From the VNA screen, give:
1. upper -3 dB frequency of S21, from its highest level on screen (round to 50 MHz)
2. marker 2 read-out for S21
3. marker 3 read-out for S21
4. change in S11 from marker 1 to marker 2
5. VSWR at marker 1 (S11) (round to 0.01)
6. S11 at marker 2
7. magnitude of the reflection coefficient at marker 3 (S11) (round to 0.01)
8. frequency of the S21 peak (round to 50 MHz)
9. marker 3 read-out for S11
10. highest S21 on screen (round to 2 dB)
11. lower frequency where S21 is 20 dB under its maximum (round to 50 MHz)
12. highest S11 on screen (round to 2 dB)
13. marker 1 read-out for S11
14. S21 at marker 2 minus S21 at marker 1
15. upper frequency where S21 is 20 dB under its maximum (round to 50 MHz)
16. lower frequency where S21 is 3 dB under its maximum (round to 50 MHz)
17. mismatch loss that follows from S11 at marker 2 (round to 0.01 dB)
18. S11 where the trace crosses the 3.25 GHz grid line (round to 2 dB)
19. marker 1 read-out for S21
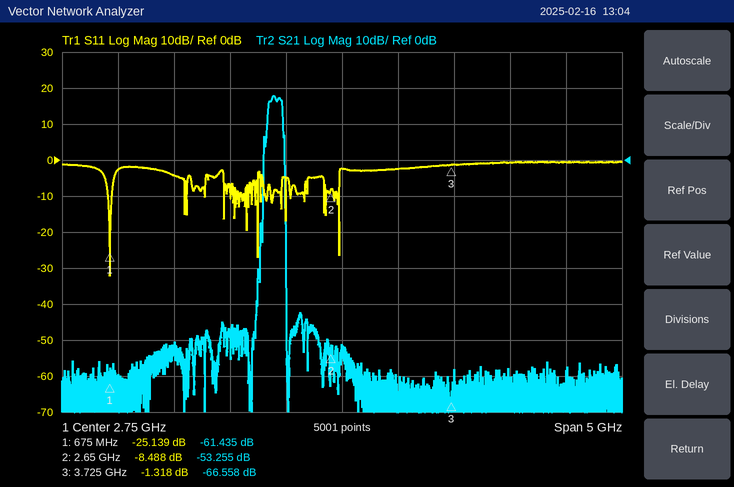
2.20 GHz
-53.255 dB
-66.558 dB
16.651 dB
1.12
-8.488 dB
0.86
2.15 GHz
-1.318 dB
18 dB
2.05 GHz
0 dB
-25.139 dB
8.180 dB
2.25 GHz
2.10 GHz
0.66 dB
-2 dB
-61.435 dB
